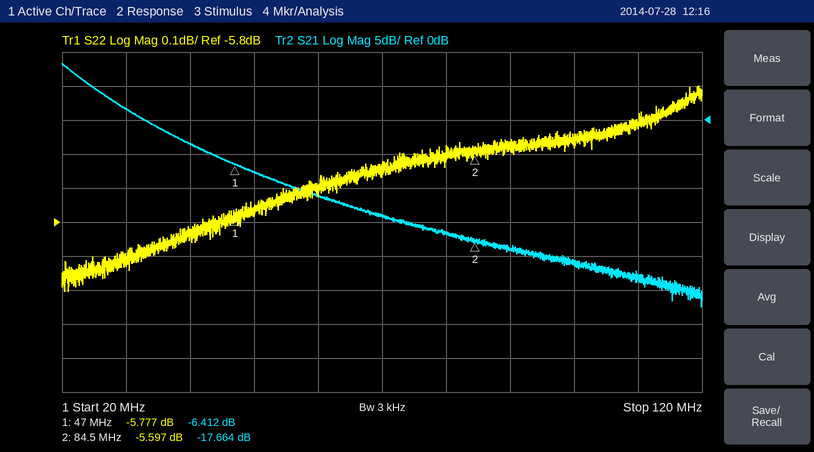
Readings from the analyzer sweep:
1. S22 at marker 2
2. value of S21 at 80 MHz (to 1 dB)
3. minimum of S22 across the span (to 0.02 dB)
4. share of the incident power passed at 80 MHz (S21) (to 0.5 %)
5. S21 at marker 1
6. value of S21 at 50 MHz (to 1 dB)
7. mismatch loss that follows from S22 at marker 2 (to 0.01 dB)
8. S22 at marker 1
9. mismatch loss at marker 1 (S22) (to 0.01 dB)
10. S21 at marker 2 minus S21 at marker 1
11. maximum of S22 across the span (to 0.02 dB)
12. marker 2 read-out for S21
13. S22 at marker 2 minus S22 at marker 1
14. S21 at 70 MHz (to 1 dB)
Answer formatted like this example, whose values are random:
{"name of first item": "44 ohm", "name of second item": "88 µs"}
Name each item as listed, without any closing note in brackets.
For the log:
{"S22 at marker 2": "-5.597 dB", "value of S21 at 80 MHz": "-17 dB", "minimum of S22 across the span": "-6.00 dB", "share of the incident power passed at 80 MHz (S21)": "2.0 %", "S21 at marker 1": "-6.412 dB", "value of S21 at 50 MHz": "-8 dB", "mismatch loss that follows from S22 at marker 2": "1.40 dB", "S22 at marker 1": "-5.777 dB", "mismatch loss at marker 1 (S22)": "1.33 dB", "S21 at marker 2 minus S21 at marker 1": "-11.252 dB", "maximum of S22 across the span": "-5.40 dB", "marker 2 read-out for S21": "-17.664 dB", "S22 at marker 2 minus S22 at marker 1": "0.180 dB", "S21 at 70 MHz": "-14 dB"}
